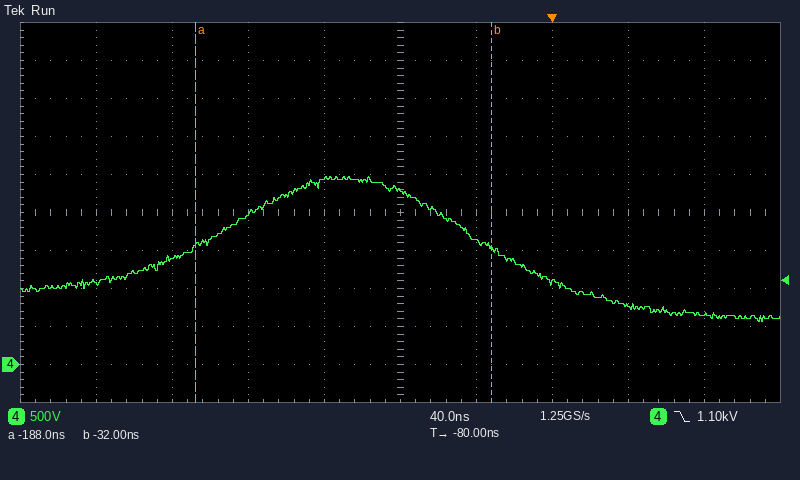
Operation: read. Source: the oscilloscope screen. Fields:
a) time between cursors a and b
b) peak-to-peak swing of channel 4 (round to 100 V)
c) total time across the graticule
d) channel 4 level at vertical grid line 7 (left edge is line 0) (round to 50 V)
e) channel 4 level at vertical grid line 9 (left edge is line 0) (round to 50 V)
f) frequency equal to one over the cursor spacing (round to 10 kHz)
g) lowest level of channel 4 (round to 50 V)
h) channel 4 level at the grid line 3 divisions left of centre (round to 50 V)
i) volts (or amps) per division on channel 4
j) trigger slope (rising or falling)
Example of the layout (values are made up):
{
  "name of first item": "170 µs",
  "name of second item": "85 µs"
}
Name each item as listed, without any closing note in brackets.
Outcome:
{
  "time between cursors a and b": "156 ns",
  "peak-to-peak swing of channel 4": "1.90 kV",
  "total time across the graticule": "400 ns",
  "channel 4 level at vertical grid line 7 (left edge is line 0)": "1.10 kV",
  "channel 4 level at vertical grid line 9 (left edge is line 0)": "650 V",
  "frequency equal to one over the cursor spacing": "6.41 MHz",
  "lowest level of channel 4": "550 V",
  "channel 4 level at the grid line 3 divisions left of centre": "1.40 kV",
  "volts (or amps) per division on channel 4": "500 V",
  "trigger slope": "falling"
}
